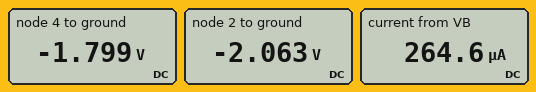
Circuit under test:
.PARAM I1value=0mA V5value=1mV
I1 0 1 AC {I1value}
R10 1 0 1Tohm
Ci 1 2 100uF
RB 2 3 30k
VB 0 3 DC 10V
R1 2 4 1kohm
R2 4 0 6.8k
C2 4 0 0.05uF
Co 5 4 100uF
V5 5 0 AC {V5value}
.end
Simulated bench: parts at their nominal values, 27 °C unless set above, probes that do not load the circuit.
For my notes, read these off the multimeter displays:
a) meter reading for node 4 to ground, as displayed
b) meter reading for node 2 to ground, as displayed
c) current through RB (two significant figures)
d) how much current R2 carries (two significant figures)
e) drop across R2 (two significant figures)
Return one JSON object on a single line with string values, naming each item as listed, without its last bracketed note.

{"meter reading for node 4 to ground, as displayed": "-1.799 V", "meter reading for node 2 to ground, as displayed": "-2.063 V", "current through RB": "260 µA", "how much current R2 carries": "260 µA", "drop across R2": "1.8 V"}
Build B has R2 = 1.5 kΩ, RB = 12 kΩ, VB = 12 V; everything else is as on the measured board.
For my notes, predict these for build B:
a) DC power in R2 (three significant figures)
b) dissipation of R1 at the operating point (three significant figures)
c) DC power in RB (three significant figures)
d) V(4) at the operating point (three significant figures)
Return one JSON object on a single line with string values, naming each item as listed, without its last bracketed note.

{"DC power in R2": "1.03 mW", "dissipation of R1 at the operating point": "685 µW", "DC power in RB": "8.22 mW", "V(4) at the operating point": "-1.24 V"}
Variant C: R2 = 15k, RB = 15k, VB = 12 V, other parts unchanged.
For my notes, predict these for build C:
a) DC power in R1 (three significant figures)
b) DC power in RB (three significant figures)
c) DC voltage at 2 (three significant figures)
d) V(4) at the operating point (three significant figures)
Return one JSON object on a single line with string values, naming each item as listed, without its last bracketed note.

{"DC power in R1": "150 µW", "DC power in RB": "2.25 mW", "DC voltage at 2": "-6.19 V", "V(4) at the operating point": "-5.81 V"}
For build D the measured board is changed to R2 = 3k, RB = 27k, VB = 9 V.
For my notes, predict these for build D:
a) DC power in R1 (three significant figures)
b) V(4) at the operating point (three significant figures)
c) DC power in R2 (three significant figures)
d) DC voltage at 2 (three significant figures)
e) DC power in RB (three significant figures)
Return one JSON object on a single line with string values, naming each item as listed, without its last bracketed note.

{"DC power in R1": "84.3 µW", "V(4) at the operating point": "-871 mV", "DC power in R2": "253 µW", "DC voltage at 2": "-1.16 V", "DC power in RB": "2.28 mW"}
